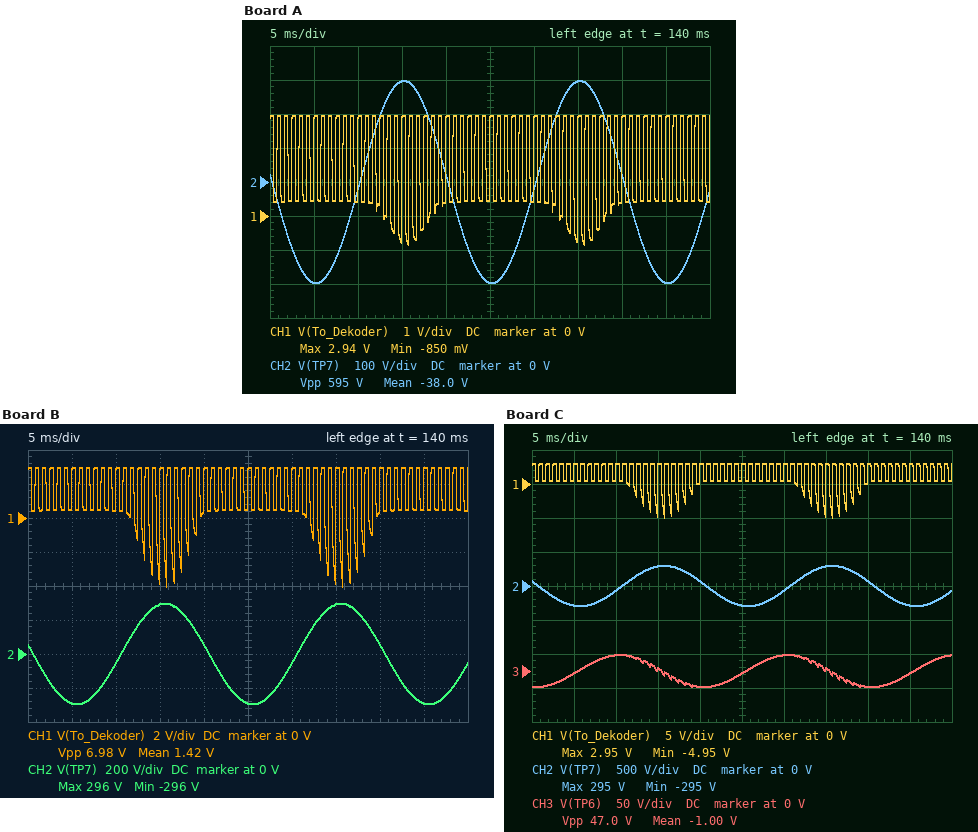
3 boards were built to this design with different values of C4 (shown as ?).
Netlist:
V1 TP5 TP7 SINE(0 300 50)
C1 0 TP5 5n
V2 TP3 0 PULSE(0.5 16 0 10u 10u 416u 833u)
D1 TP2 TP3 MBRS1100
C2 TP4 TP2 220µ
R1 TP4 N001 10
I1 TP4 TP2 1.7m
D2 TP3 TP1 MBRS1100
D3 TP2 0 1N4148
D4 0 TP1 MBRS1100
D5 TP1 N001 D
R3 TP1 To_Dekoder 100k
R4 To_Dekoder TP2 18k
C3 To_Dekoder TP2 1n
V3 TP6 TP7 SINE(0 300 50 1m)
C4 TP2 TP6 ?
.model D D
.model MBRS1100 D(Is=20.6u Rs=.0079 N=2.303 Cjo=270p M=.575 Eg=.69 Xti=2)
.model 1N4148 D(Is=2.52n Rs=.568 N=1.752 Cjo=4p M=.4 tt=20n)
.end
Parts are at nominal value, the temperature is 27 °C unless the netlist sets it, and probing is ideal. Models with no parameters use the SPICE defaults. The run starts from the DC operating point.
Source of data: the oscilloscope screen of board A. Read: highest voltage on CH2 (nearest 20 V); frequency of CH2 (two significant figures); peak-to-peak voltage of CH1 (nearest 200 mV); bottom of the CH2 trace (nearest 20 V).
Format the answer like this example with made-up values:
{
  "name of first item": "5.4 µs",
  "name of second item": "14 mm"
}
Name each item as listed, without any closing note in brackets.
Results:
{
  "highest voltage on CH2": "300 V",
  "frequency of CH2": "50 Hz",
  "peak-to-peak voltage of CH1": "3.8 V",
  "bottom of the CH2 trace": "-300 V"
}
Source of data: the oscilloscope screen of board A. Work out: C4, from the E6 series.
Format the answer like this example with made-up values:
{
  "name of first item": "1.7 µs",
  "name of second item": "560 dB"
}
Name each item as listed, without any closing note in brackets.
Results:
{
  "C4, from the E6 series": "1.5 nF"
}
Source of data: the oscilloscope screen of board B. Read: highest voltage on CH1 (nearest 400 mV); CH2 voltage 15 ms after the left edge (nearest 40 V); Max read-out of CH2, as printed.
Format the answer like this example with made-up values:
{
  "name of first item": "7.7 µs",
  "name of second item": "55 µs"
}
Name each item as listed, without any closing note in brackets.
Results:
{
  "highest voltage on CH1": "2.8 V",
  "CH2 voltage 15 ms after the left edge": "280 V",
  "Max read-out of CH2, as printed": "296 V"
}
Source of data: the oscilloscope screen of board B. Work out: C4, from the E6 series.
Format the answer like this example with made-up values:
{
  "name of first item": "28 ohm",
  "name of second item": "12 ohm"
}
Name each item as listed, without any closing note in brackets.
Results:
{
  "C4, from the E6 series": "6.8 nF"
}
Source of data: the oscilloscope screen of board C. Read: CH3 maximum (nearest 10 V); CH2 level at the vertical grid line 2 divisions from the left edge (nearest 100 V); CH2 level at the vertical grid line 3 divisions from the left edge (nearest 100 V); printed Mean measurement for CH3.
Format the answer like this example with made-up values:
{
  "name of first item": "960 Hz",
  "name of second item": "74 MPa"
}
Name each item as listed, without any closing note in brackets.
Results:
{
  "CH3 maximum": "20 V",
  "CH2 level at the vertical grid line 2 divisions from the left edge": "-100 V",
  "CH2 level at the vertical grid line 3 divisions from the left edge": "300 V",
  "printed Mean measurement for CH3": "-1.00 V"
}
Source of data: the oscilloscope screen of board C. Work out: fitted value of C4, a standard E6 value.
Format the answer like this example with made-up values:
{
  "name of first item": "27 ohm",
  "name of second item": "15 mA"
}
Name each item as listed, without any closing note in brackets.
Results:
{
  "fitted value of C4, a standard E6 value": "15 nF"
}
